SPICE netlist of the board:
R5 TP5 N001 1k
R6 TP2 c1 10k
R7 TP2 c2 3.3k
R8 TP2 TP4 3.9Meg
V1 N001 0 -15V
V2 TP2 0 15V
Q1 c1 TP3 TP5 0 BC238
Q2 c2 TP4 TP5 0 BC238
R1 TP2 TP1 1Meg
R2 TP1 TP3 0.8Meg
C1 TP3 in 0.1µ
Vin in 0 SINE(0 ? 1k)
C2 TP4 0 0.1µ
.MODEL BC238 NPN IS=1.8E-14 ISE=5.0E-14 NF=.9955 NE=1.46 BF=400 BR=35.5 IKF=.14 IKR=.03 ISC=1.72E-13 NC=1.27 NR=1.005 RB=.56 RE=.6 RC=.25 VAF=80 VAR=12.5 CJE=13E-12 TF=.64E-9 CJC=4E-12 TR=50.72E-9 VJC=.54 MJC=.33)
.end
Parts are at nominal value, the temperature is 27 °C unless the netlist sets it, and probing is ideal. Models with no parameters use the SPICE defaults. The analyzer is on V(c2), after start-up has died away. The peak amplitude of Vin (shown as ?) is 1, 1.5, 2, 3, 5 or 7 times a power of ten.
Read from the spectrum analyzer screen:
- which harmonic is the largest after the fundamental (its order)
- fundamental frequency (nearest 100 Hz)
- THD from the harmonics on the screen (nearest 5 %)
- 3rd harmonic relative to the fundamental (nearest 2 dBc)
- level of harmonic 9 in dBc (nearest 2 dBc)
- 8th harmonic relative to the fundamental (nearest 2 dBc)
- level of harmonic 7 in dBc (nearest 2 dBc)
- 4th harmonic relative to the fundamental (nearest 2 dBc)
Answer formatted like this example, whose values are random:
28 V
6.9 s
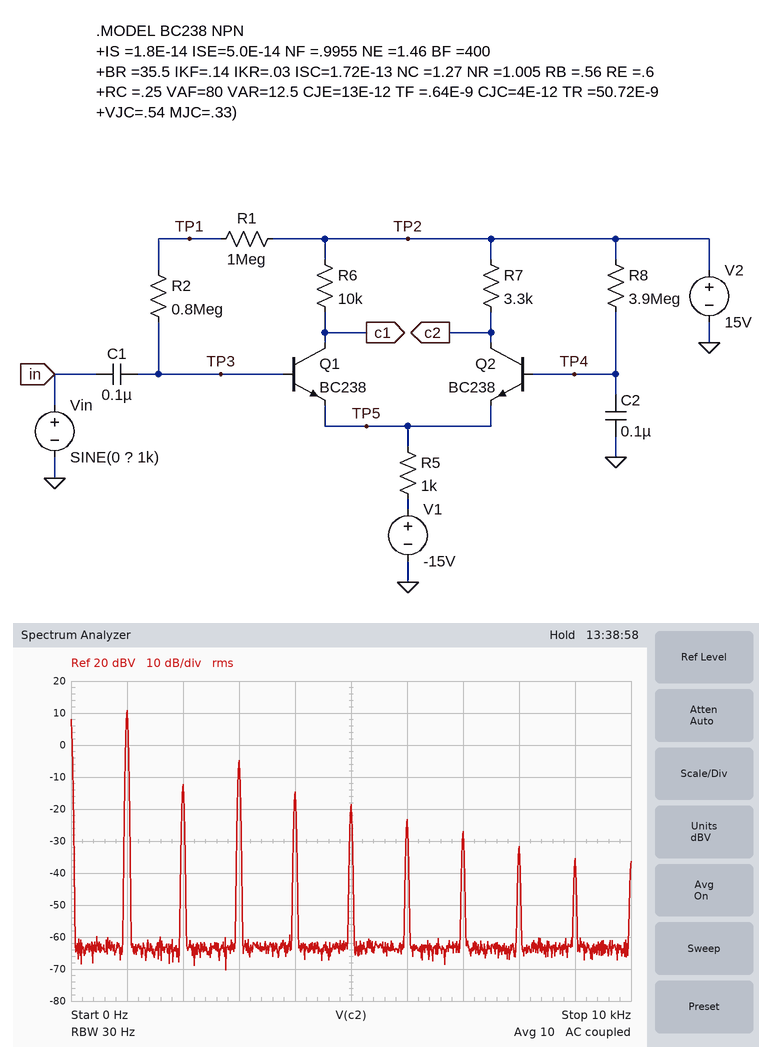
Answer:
3
1.0 kHz
20 %
-16 dBc
-46 dBc
-42 dBc
-38 dBc
-26 dBc
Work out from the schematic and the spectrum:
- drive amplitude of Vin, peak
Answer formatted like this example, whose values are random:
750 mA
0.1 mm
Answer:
100 mV
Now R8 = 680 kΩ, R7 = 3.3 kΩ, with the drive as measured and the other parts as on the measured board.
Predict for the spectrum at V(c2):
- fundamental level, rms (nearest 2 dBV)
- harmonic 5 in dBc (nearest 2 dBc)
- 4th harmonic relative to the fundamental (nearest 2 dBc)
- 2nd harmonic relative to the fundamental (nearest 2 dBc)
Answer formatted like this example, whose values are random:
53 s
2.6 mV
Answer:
8 dBV
-32 dBc
-20 dBc
-14 dBc
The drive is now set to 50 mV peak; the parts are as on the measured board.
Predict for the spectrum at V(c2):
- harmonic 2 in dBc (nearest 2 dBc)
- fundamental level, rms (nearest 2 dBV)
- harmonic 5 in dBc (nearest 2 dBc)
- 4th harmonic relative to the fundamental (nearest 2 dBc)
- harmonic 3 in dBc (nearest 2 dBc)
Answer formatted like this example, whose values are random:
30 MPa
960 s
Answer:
-14 dBc
6 dBV
-32 dBc
-30 dBc
-20 dBc
